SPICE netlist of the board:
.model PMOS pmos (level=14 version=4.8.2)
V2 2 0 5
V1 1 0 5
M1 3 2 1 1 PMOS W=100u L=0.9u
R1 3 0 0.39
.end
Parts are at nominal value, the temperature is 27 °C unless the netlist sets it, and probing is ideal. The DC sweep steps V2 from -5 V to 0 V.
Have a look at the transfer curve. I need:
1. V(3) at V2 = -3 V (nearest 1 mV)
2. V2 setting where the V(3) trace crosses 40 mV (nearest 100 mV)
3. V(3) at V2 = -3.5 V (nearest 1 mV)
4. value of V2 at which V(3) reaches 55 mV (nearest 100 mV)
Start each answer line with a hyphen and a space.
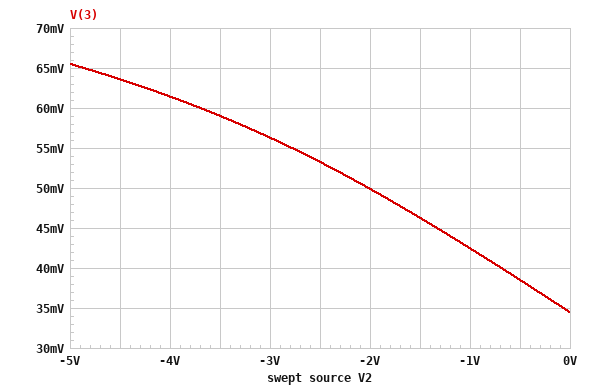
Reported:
- 56 mV
- -700 mV
- 59 mV
- -2.8 V
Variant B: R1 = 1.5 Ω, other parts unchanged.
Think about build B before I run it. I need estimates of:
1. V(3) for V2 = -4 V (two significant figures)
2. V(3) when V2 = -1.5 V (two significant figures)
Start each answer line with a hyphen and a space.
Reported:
- 230 mV
- 180 mV
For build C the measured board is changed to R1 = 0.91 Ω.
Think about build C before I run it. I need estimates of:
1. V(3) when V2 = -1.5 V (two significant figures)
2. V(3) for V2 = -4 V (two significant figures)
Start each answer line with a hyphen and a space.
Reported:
- 110 mV
- 140 mV
